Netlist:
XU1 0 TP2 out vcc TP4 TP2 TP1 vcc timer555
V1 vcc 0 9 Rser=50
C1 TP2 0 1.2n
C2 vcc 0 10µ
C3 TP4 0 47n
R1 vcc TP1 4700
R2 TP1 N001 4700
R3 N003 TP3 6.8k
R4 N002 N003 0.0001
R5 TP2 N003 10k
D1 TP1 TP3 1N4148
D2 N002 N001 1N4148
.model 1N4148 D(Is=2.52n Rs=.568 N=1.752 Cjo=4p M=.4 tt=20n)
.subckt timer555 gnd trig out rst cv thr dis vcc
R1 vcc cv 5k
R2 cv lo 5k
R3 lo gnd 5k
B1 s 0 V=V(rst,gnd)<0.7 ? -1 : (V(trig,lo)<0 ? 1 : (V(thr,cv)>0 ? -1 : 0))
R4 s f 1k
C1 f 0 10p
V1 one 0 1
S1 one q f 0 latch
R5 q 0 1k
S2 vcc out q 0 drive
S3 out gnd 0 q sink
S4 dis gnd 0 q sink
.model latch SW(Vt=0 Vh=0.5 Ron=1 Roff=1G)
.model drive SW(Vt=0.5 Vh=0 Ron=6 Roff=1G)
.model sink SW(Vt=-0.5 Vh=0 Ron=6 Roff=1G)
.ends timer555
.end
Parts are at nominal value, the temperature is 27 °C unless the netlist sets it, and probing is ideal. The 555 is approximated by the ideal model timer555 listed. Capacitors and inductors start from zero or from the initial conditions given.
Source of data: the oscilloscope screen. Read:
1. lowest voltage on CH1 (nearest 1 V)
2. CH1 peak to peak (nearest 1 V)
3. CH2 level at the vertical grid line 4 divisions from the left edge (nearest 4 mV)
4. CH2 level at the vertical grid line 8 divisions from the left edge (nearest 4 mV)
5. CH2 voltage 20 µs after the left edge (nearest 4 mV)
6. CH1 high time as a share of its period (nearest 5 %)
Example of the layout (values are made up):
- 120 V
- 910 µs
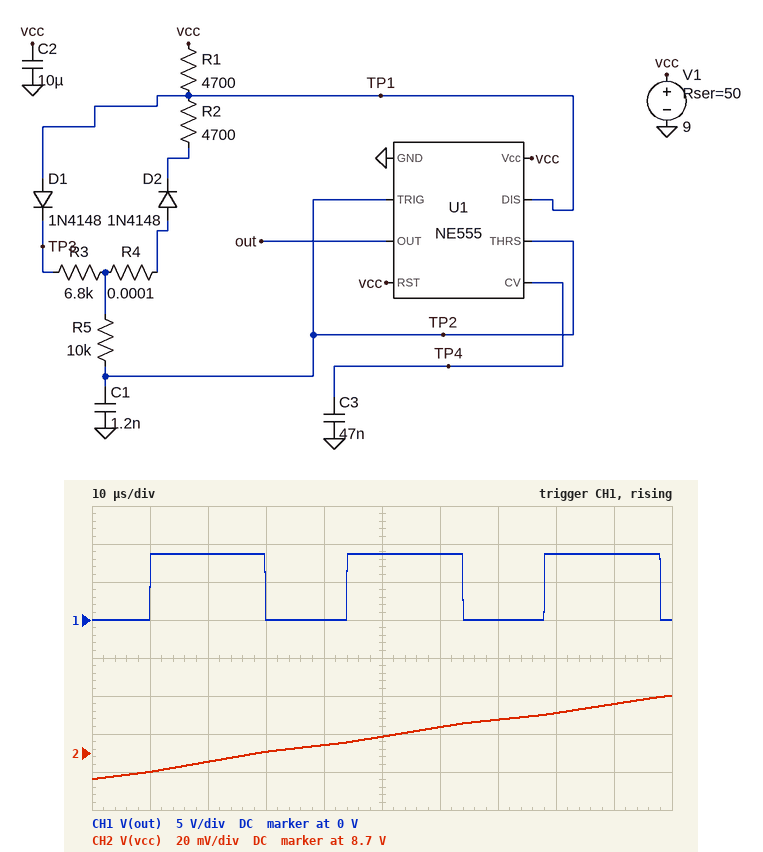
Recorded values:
- 0 V
- 9 V
- 8.704 V
- 8.720 V
- 8.696 V
- 60 %
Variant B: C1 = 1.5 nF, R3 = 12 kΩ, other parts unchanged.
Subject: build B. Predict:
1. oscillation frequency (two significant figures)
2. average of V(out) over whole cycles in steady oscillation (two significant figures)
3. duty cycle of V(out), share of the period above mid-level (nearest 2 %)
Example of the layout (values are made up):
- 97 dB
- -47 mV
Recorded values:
- 21 kHz
- 5.6 V
- 64 %
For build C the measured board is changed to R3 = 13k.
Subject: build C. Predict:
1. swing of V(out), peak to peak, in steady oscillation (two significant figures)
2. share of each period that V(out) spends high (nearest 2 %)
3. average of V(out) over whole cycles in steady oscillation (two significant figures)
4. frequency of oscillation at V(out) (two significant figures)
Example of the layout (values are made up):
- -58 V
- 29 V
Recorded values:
- 8.8 V
- 64 %
- 5.6 V
- 25 kHz
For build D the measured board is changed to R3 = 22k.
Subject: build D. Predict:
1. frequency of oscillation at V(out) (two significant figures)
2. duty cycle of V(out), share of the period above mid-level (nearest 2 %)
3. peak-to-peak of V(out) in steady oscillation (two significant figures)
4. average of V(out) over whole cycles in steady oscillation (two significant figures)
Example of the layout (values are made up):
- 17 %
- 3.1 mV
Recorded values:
- 21 kHz
- 70 %
- 8.8 V
- 6.2 V
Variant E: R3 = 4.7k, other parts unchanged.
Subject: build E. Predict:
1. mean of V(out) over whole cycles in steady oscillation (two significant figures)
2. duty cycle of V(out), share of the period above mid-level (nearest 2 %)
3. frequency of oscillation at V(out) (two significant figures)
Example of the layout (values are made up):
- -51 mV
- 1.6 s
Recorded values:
- 4.9 V
- 56 %
- 31 kHz
